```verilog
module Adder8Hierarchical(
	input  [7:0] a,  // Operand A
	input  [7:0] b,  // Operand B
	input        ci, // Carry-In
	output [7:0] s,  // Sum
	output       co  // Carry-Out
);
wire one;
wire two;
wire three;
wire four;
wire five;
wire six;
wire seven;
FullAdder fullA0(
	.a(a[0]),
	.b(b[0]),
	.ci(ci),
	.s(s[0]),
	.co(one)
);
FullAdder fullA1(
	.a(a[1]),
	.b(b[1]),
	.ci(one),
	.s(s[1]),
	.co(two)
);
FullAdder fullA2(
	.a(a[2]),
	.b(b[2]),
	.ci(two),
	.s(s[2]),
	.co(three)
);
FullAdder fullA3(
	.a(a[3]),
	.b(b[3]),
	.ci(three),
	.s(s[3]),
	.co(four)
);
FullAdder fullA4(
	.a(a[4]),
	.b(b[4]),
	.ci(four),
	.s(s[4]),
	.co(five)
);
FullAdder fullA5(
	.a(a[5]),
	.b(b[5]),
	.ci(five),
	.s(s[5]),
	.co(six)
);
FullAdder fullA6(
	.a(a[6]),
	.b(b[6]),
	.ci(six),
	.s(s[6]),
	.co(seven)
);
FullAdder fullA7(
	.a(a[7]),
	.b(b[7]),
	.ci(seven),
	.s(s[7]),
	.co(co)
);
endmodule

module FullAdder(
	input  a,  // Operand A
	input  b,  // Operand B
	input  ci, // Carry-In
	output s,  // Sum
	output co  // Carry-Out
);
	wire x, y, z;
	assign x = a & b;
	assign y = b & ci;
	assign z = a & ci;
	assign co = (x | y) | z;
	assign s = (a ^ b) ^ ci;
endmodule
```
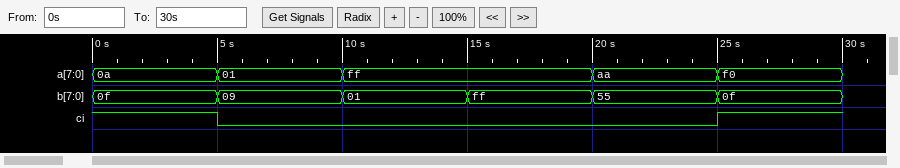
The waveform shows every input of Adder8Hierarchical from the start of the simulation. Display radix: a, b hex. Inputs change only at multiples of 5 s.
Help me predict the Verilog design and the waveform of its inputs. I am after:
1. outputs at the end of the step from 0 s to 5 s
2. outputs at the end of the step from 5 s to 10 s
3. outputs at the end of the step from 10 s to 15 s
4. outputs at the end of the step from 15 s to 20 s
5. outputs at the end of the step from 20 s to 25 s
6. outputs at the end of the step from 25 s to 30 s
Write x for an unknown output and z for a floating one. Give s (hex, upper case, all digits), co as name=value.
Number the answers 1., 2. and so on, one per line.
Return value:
1. s=1A, co=0
2. s=0A, co=0
3. s=00, co=1
4. s=FE, co=1
5. s=FF, co=0
6. s=00, co=1
